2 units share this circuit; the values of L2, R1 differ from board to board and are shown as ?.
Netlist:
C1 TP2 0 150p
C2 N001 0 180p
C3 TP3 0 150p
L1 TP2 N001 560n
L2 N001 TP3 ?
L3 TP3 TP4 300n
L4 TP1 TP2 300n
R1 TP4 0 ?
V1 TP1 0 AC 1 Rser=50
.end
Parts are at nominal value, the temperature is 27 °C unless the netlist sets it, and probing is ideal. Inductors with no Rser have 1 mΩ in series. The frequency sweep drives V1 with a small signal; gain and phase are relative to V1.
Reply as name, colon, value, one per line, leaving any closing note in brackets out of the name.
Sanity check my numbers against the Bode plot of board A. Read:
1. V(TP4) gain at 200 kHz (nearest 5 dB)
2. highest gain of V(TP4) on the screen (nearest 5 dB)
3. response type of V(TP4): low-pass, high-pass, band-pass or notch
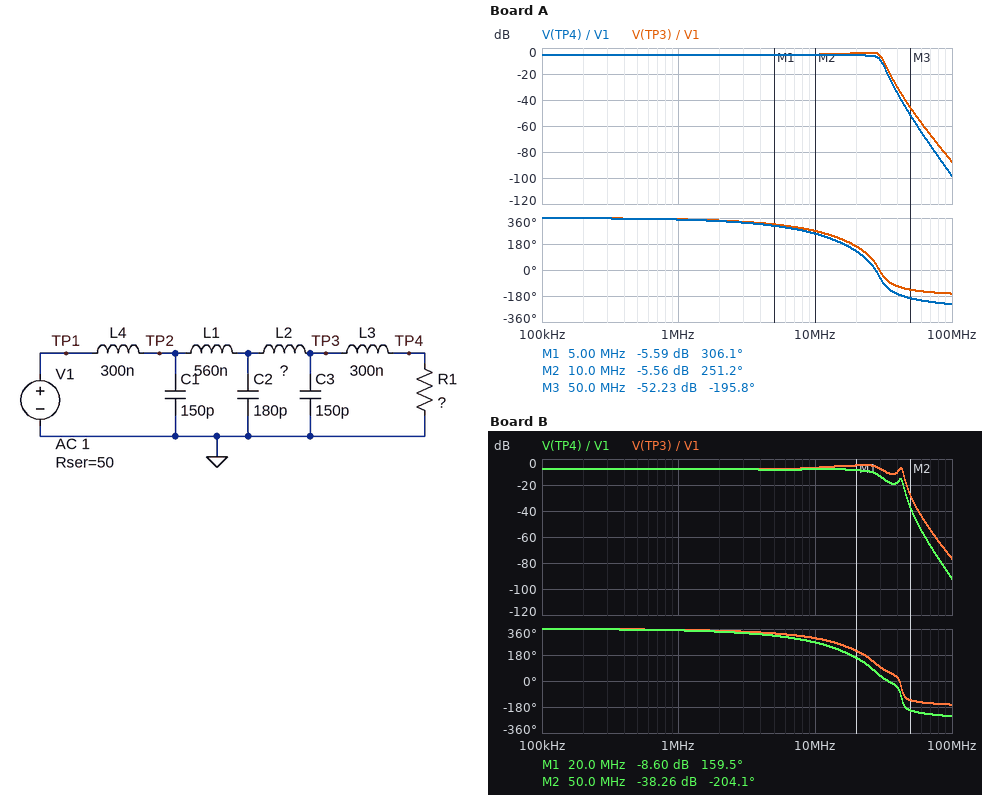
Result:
V(TP4) gain at 200 kHz: -5 dB
highest gain of V(TP4) on the screen: -5 dB
response type of V(TP4): low-pass, high-pass, band-pass or notch: low-pass
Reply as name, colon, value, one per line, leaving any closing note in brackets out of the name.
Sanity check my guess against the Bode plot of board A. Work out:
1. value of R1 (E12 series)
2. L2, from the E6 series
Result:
value of R1: 56 Ω
L2, from the E6 series: 680 nH
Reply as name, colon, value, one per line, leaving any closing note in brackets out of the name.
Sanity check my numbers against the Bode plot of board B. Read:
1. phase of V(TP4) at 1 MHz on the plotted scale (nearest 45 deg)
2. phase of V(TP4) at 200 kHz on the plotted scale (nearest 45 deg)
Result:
phase of V(TP4) at 1 MHz on the plotted scale: 360 deg
phase of V(TP4) at 200 kHz on the plotted scale: 360 deg
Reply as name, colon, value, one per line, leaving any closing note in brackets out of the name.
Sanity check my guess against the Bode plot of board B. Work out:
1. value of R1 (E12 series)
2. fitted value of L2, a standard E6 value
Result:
value of R1: 33 Ω
fitted value of L2, a standard E6 value: 220 nH
